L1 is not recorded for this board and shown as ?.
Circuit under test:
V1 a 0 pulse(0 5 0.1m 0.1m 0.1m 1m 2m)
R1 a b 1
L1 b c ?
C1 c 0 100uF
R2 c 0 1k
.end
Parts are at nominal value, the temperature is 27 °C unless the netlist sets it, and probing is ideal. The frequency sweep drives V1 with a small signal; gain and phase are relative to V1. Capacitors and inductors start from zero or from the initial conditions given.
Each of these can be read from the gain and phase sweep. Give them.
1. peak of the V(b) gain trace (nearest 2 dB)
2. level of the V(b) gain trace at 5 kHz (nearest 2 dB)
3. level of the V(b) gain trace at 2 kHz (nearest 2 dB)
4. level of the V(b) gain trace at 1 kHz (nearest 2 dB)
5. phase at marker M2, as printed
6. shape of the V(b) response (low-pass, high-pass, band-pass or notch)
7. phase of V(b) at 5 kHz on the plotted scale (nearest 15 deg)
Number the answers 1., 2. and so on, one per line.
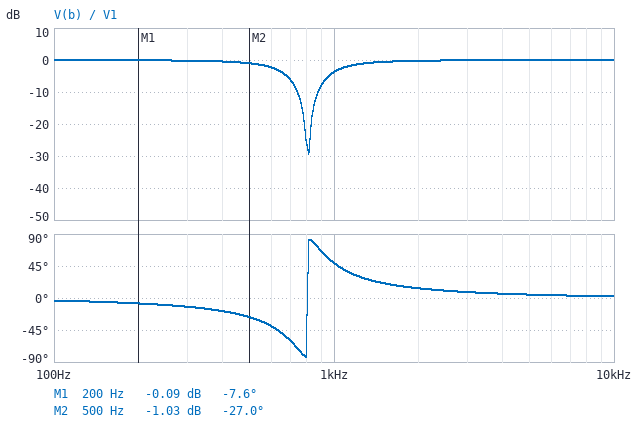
1. 0 dB
2. 0 dB
3. 0 dB
4. -4 dB
5. -27.0 deg
6. notch
7. 0 deg
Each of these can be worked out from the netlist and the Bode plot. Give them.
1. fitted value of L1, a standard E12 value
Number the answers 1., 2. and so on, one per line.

1. 390 µH
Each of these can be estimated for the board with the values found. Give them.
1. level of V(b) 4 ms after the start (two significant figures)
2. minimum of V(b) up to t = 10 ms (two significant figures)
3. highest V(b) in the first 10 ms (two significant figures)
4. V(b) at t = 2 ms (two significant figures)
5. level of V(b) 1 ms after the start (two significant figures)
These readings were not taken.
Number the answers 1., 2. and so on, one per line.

1. -520 mV
2. -710 mV
3. 5.9 V
4. -580 mV
5. 5.7 V
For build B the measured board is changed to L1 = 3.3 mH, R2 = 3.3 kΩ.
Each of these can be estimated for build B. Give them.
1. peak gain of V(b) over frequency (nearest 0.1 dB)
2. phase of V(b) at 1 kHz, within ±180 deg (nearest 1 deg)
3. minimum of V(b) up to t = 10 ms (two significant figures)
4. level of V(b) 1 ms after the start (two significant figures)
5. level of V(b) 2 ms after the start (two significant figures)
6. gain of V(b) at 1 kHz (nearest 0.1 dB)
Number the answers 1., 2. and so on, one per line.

1. 0 dB
2. 3 deg
3. -590 mV
4. 4.2 V
5. 790 mV
6. 0 dB
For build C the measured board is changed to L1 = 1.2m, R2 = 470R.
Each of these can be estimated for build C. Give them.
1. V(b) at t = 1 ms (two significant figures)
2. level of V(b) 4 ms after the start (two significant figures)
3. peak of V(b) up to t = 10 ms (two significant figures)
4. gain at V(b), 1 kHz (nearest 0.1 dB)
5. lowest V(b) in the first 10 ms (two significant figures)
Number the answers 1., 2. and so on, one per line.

1. 4.3 V
2. 2.2 V
3. 6.4 V
4. -0.1 dB
5. -690 mV
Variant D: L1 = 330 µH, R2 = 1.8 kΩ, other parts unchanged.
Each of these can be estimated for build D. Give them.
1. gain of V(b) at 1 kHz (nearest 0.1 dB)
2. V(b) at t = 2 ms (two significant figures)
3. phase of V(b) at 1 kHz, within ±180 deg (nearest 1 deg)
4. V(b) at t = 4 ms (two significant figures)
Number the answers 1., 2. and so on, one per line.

1. -7.3 dB
2. -600 mV
3. 64 deg
4. -570 mV
